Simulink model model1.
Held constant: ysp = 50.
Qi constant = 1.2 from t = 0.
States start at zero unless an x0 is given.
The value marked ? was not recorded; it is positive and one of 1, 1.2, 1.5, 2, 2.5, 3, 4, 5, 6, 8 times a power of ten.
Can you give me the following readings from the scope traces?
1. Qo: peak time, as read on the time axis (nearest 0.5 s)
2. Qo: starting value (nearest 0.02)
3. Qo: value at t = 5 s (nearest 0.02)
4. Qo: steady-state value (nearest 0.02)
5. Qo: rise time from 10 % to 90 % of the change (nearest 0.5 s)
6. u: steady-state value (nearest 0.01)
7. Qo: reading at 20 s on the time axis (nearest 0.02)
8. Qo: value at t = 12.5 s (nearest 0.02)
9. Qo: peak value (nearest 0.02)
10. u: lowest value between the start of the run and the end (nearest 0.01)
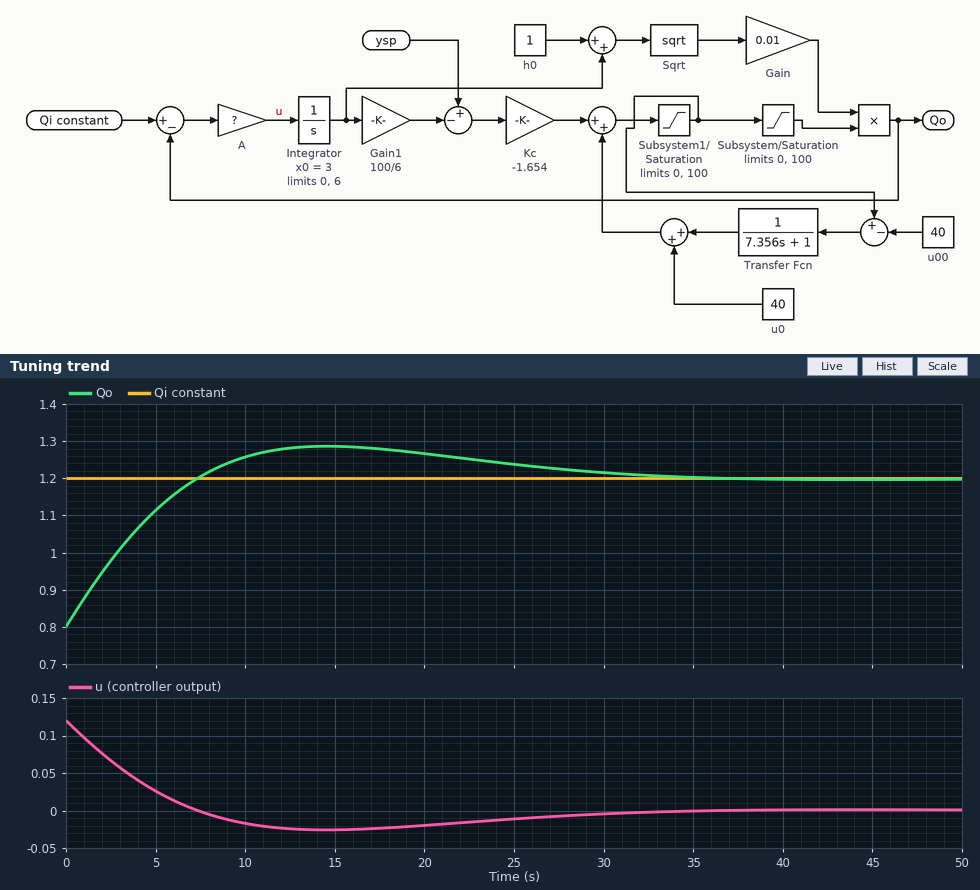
14.5 s
0.80
1.12
1.20
5.5 s
0.00
1.26
1.28
1.28
-0.03
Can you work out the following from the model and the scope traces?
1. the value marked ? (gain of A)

0.3
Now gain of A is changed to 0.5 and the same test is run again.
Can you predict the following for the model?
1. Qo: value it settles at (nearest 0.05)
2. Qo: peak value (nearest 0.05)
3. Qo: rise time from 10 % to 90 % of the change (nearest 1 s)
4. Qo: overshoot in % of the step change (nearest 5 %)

1.20
1.25
4 s
15 %
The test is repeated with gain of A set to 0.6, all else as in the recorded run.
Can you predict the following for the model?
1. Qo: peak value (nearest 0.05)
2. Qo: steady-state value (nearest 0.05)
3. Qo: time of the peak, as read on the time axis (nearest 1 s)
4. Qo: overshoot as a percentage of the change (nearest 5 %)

1.25
1.20
9 s
15 %
